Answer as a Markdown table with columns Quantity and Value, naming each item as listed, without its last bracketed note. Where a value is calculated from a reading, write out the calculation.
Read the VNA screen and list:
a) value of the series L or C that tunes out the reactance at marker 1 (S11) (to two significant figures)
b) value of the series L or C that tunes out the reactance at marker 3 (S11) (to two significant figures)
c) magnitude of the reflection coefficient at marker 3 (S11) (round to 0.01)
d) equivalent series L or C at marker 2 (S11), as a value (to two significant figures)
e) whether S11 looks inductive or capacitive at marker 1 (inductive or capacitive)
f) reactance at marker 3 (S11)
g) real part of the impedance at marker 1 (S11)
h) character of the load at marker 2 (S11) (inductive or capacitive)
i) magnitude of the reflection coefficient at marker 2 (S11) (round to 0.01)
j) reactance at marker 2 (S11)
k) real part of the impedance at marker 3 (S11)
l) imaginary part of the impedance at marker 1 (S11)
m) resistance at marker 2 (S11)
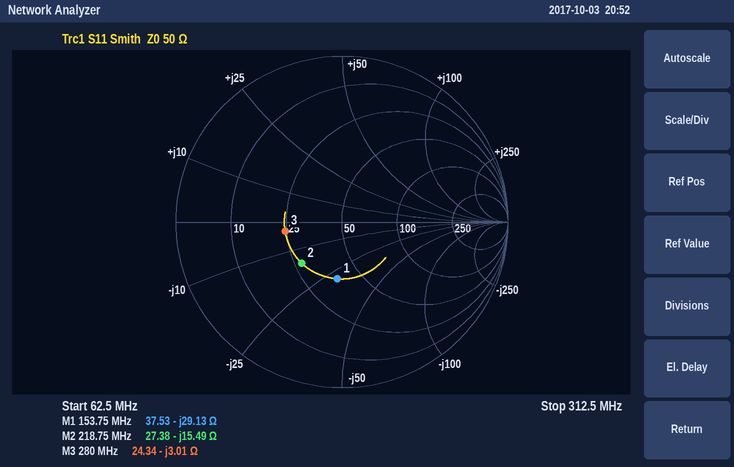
| Quantity | Value |
|---|---|
| value of the series L or C that tunes out the reactance at marker 1 (S11) | L = 29.13 Ω/(2π × 153.75 MHz) ≈ 30 nH |
| value of the series L or C that tunes out the reactance at marker 3 (S11) | L = 3.01 Ω/(2π × 280 MHz) ≈ 1.7 nH |
| magnitude of the reflection coefficient at marker 3 (S11) | 0.35 |
| equivalent series L or C at marker 2 (S11), as a value | C = 1/(2π × 218.75 MHz × 15.49 Ω) ≈ 47 pF |
| whether S11 looks inductive or capacitive at marker 1 | capacitive |
| reactance at marker 3 | -3.01 Ω |
| real part of the impedance at marker 1 | 37.53 Ω |
| character of the load at marker 2 (S11) | capacitive |
| magnitude of the reflection coefficient at marker 2 (S11) | 0.35 |
| reactance at marker 2 | -15.49 Ω |
| real part of the impedance at marker 3 | 24.34 Ω |
| imaginary part of the impedance at marker 1 | -29.13 Ω |
| resistance at marker 2 | 27.38 Ω |
